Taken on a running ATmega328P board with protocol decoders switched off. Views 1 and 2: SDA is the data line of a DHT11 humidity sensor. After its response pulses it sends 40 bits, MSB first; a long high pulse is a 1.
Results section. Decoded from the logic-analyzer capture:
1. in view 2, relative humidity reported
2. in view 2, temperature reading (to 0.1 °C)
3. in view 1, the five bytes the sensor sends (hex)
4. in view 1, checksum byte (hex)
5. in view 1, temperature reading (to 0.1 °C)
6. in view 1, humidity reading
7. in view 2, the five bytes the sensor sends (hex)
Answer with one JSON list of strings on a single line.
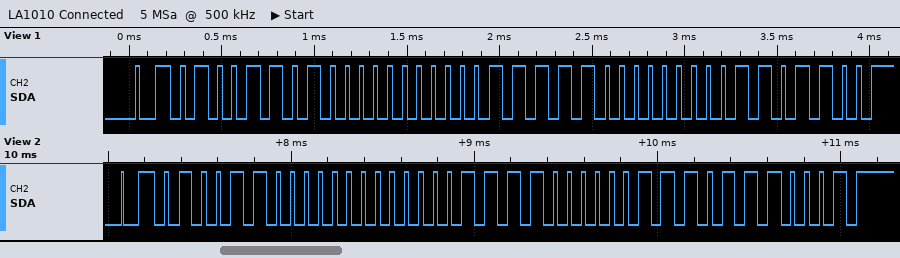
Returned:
["76 %", "30.7 °C", "4D 00 1F 00 6C", "0x6C", "31.0 °C", "77 %", "4C 00 1E 07 71"]
